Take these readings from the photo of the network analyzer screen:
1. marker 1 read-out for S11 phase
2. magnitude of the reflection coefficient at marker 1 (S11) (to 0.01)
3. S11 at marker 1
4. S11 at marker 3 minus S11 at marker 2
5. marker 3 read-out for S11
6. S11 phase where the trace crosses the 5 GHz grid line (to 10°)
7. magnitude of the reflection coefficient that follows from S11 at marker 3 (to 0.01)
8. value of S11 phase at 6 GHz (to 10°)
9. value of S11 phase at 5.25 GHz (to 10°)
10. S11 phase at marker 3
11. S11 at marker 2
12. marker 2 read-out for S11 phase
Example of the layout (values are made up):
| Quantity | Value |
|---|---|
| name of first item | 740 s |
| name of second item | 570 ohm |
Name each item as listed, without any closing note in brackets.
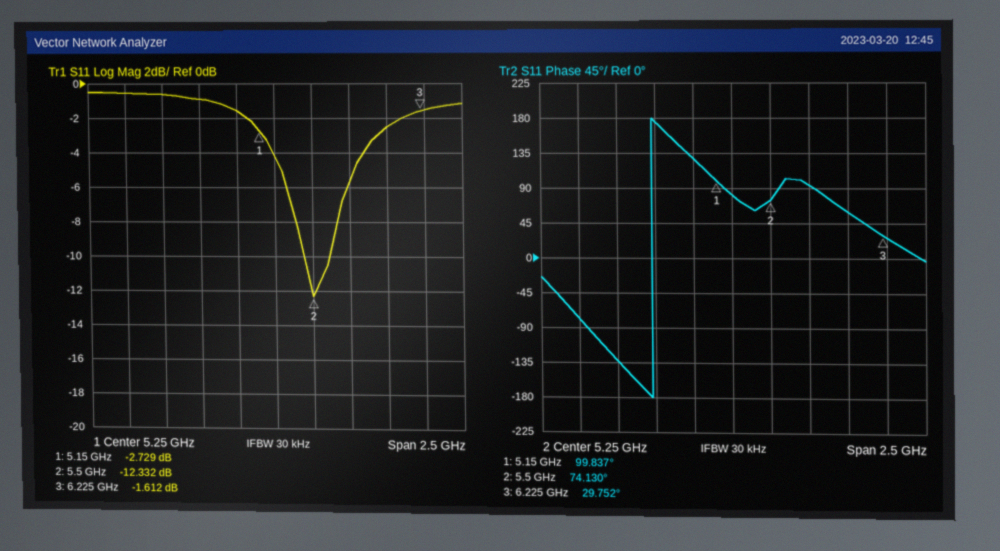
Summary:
| Quantity | Value |
|---|---|
| marker 1 read-out for S11 phase | 99.837° |
| magnitude of the reflection coefficient at marker 1 (S11) | 0.73 |
| S11 at marker 1 | -2.729 dB |
| S11 at marker 3 minus S11 at marker 2 | 10.720 dB |
| marker 3 read-out for S11 | -1.612 dB |
| S11 phase where the trace crosses the 5 GHz grid line | 130° |
| magnitude of the reflection coefficient that follows from S11 at marker 3 | 0.83 |
| value of S11 phase at 6 GHz | 60° |
| value of S11 phase at 5.25 GHz | 80° |
| S11 phase at marker 3 | 29.752° |
| S11 at marker 2 | -12.332 dB |
| marker 2 read-out for S11 phase | 74.130° |
